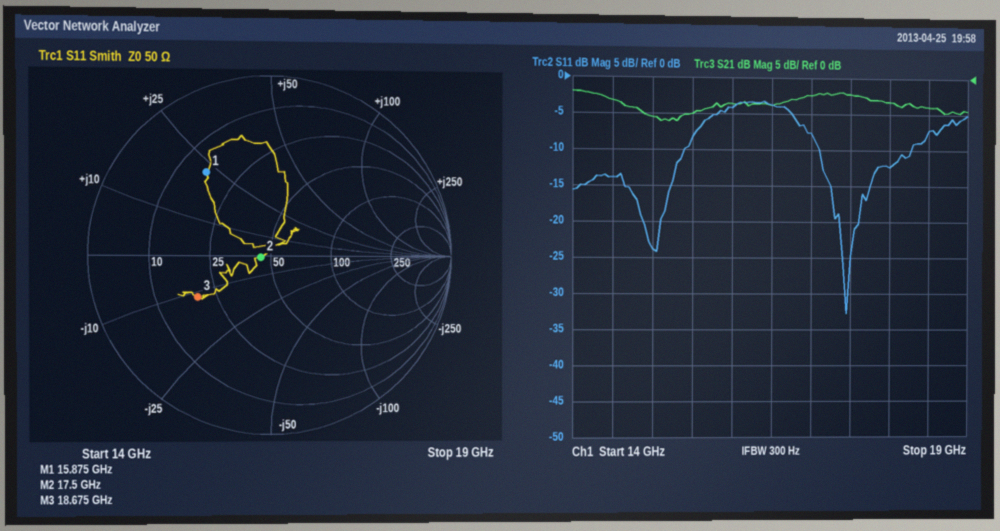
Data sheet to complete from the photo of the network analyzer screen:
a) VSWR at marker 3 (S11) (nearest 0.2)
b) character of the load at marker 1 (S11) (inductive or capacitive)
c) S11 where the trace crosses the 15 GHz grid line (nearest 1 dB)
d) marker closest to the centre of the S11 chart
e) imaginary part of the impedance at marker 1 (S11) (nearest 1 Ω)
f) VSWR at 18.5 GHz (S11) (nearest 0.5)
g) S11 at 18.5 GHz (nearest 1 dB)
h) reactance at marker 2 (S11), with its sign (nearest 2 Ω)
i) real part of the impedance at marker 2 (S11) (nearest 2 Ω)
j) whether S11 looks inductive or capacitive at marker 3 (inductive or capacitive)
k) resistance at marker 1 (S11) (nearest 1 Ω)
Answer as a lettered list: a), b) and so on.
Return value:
a) 2.8
b) inductive
c) -24 dB
d) marker 2
e) +23 Ω
f) 2.5
g) -7 dB
h) 0 Ω
i) 44 Ω
j) capacitive
k) 16 Ω
